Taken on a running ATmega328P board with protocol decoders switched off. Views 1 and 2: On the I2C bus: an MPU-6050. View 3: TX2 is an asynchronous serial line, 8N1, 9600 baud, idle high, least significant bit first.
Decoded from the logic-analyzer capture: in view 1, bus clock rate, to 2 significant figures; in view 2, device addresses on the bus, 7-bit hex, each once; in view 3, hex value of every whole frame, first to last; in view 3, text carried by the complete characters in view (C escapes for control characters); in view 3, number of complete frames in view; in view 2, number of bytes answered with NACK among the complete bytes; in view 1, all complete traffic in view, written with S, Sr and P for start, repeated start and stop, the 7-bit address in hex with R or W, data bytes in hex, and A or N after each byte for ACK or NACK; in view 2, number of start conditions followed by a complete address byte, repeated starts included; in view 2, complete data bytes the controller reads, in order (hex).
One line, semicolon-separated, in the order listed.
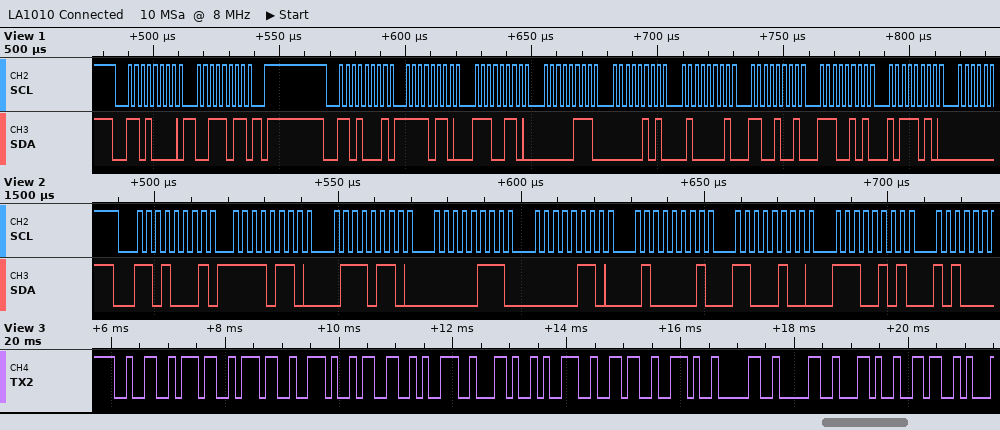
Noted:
400 kHz; 0x68; 32 37 37 2E 33 39 2C 39 36 2E 30 30 2C 36; "277.39,96.00,6"; 14; 0; S 68W A 3B A P S 68R A F6 A E6 A 07 A 05 A 41 A C9 A E5 A BA A; 1; F6 76 07 06 41 C4 E5
